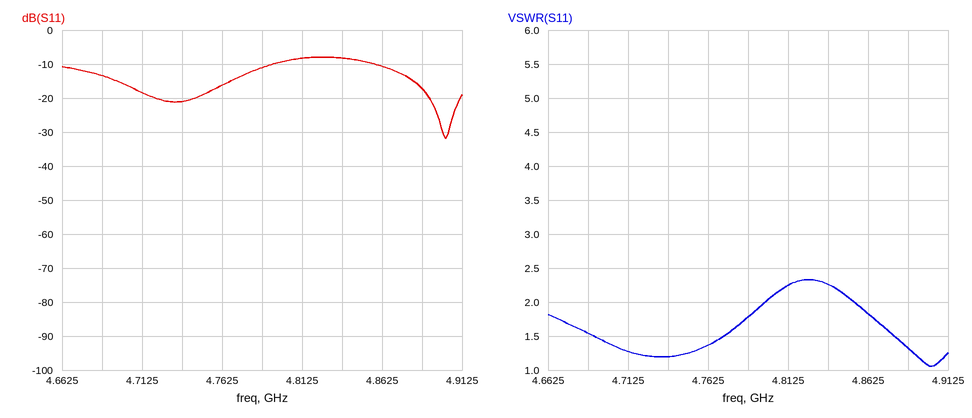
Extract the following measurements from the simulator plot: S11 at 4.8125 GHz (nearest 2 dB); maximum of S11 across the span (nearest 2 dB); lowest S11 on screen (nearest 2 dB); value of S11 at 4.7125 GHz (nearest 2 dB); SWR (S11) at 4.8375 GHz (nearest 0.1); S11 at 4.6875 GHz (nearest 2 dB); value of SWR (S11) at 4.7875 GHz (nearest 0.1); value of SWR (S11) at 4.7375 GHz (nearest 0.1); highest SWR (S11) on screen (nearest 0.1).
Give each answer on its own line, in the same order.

-8 dB
-8 dB
-32 dB
-18 dB
2.3
-14 dB
1.8
1.2
2.3
